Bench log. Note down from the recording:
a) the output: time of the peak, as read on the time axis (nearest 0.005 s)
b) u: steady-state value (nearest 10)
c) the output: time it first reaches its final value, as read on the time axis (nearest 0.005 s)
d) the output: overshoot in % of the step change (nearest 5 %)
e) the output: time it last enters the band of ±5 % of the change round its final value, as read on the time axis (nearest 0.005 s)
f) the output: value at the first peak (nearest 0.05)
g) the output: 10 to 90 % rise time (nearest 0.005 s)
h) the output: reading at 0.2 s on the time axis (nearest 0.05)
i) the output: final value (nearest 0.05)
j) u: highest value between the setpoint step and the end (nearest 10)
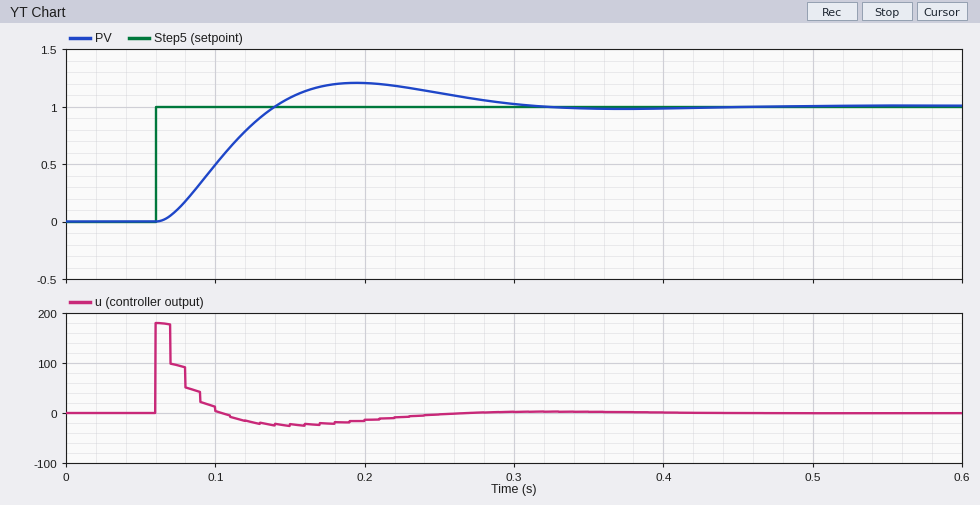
0.195 s
0
0.140 s
20 %
0.280 s
1.20
0.055 s
1.20
1.00
180
